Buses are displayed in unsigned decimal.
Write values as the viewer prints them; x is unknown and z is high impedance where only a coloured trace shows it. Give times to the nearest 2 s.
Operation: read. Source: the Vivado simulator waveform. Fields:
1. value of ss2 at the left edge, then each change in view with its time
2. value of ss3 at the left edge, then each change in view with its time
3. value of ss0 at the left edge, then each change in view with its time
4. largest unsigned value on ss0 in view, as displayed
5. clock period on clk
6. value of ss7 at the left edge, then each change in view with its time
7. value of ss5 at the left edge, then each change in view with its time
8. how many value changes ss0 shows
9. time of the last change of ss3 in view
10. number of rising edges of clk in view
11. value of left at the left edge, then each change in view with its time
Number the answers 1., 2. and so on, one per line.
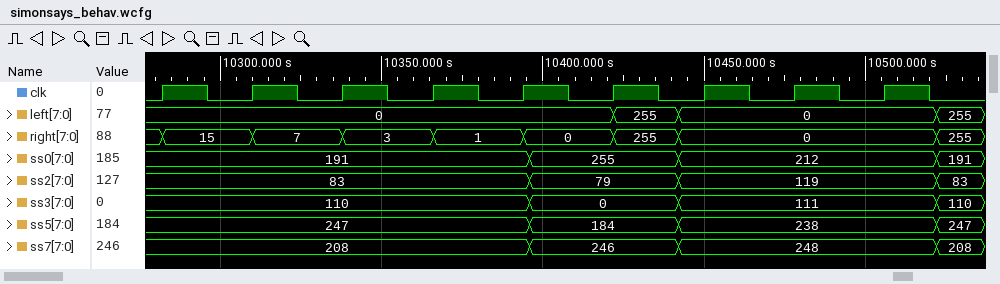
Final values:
1. 83, 79 at 10396 s, 119 at 10442 s, 83 at 10522 s
2. 110, 0 at 10396 s, 111 at 10442 s, 110 at 10522 s
3. 191, 255 at 10396 s, 212 at 10442 s, 191 at 10522 s
4. 255
5. 28 s
6. 208, 246 at 10396 s, 248 at 10442 s, 208 at 10522 s
7. 247, 184 at 10396 s, 238 at 10442 s, 247 at 10522 s
8. 3
9. 10522 s
10. 9
11. 0, 255 at 10422 s, 0 at 10442 s, 255 at 10522 s
